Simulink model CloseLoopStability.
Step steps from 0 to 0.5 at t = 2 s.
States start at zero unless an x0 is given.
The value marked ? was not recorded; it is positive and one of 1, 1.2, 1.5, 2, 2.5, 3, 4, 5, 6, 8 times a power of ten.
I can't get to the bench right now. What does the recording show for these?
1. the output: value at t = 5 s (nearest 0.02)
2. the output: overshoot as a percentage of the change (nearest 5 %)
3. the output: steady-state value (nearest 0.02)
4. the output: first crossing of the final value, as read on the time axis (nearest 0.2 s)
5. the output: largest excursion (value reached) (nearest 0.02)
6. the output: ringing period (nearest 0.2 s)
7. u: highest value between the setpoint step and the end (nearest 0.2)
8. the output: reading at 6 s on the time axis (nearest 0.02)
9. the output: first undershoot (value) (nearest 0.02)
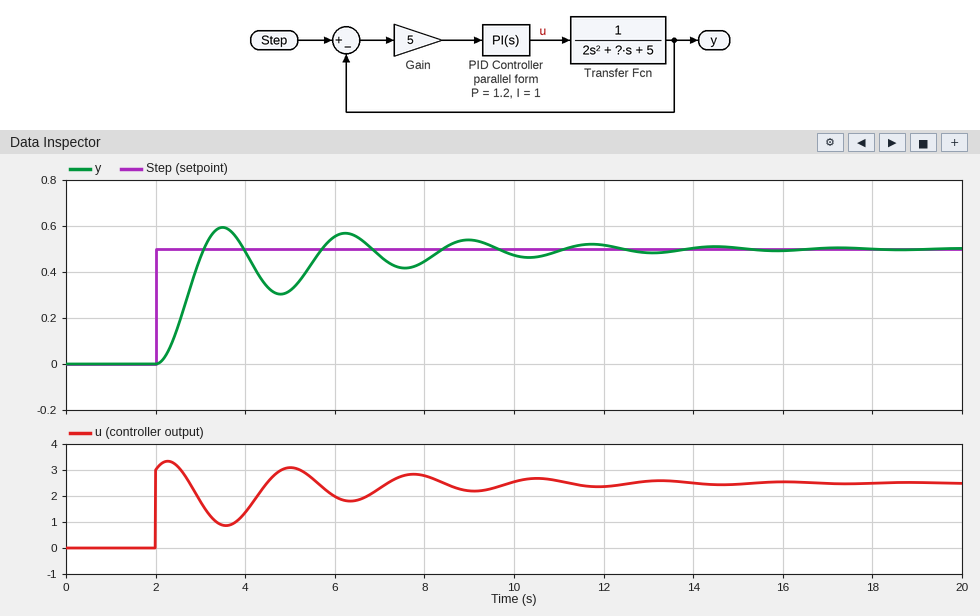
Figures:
0.32
20 %
0.50
3.0 s
0.60
2.8 s
3.4
0.56
0.30
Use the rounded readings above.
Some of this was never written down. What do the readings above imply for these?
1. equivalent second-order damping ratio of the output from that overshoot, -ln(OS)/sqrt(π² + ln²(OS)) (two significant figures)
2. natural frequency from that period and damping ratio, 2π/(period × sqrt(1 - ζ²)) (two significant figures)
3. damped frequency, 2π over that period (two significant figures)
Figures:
0.46
2.5 rad/s
2.2 rad/s
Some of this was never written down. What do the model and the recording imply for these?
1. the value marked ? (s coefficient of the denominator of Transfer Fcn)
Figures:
2
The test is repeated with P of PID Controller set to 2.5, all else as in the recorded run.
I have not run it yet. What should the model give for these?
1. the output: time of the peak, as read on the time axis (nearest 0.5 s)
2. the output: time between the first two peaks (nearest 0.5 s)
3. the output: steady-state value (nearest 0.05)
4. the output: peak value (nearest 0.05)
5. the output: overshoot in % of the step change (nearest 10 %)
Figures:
3.0 s
2.0 s
0.50
0.65
30 %
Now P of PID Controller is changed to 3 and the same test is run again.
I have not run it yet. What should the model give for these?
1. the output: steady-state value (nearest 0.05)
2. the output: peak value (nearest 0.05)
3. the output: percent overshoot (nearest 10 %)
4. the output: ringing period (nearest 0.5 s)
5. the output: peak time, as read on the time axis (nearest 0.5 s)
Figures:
0.50
0.65
30 %
2.0 s
3.0 s
